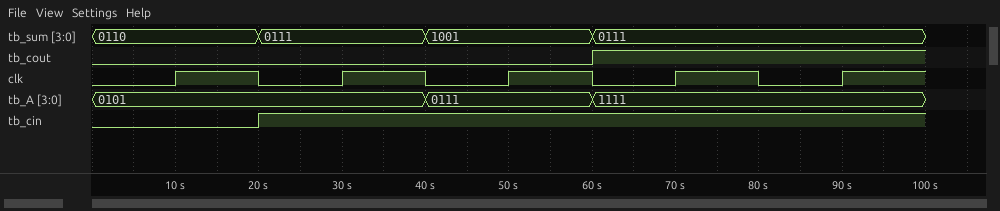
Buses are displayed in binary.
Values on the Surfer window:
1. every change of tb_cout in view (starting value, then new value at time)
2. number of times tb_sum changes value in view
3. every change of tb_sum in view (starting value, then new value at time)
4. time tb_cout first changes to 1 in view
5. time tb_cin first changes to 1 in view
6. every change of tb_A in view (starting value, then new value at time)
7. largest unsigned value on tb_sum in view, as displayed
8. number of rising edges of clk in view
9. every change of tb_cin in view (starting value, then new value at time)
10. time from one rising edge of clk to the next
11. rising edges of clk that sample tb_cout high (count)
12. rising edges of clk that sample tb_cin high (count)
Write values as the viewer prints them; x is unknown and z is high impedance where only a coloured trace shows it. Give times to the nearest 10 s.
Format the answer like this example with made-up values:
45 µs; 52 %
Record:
0, 1 at 60 s; 3; 0110, 0111 at 20 s, 1001 at 40 s, 0111 at 60 s; 60 s; 20 s; 0101, 0111 at 40 s, 1111 at 60 s; 1001; 5; 0, 1 at 20 s; 20 s; 2; 4
